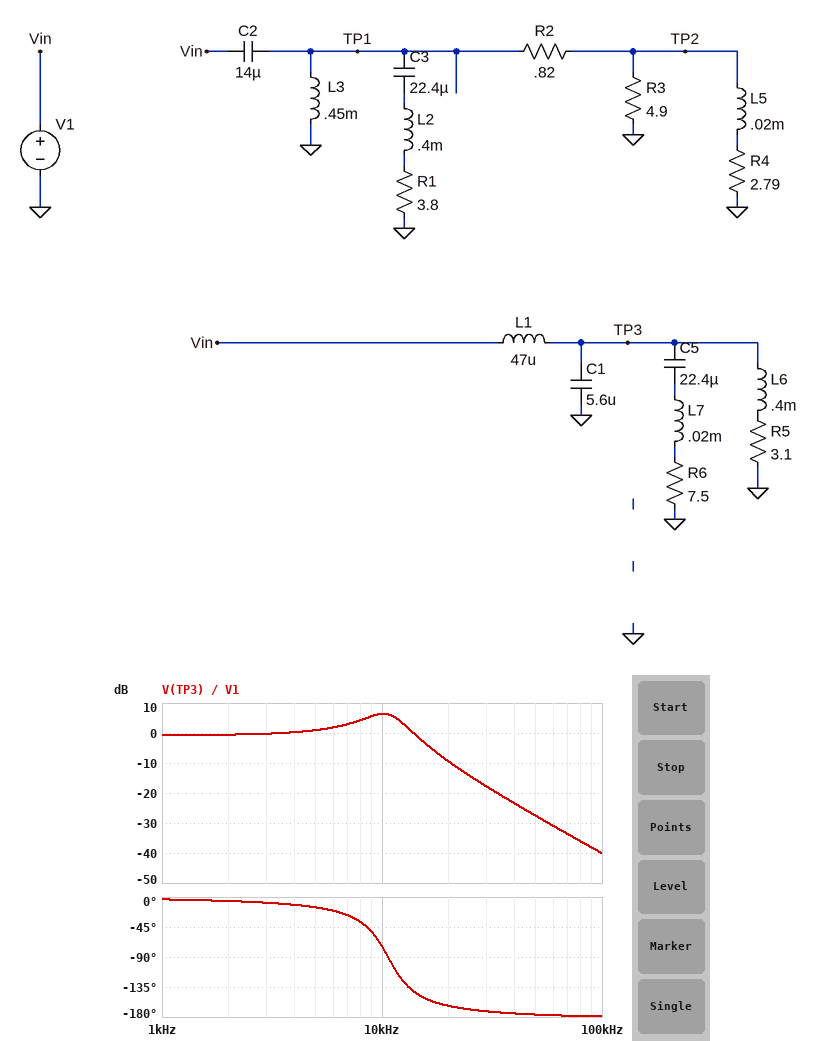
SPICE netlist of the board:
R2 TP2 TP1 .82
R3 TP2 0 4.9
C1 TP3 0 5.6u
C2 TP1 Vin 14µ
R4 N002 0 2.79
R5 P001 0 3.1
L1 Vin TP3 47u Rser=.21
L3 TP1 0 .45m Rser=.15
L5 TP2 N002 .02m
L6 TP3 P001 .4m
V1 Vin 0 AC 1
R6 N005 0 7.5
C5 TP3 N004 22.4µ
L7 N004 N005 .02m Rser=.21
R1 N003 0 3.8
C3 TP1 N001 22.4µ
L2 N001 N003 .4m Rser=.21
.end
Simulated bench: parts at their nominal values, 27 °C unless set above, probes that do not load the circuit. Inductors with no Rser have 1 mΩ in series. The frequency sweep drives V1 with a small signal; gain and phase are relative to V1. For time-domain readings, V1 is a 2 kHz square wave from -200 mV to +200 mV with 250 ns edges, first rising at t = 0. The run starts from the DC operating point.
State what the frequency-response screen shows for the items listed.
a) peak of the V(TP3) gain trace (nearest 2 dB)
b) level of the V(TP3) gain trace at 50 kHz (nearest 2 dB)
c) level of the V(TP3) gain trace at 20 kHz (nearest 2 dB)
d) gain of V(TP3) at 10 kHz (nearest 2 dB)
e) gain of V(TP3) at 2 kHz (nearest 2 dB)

6 dB
-28 dB
-10 dB
6 dB
0 dB
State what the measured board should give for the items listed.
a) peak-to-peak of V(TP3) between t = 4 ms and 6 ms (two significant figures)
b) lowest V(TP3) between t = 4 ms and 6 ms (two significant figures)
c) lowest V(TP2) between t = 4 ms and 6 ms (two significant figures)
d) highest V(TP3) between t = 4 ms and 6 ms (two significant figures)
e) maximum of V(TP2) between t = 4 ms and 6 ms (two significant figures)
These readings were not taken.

720 mV
-360 mV
-340 mV
360 mV
340 mV
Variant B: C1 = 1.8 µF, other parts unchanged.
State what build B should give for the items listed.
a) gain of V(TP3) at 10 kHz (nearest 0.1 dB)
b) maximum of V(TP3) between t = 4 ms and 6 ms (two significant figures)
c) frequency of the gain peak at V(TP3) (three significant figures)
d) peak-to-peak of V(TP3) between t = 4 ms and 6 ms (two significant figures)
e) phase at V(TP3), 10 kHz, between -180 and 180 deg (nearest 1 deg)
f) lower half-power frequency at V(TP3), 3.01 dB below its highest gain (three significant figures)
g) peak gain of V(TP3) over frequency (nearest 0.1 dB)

0.6 dB
290 mV
18.0 kHz
580 mV
-26 deg
6.71 kHz
2.8 dB
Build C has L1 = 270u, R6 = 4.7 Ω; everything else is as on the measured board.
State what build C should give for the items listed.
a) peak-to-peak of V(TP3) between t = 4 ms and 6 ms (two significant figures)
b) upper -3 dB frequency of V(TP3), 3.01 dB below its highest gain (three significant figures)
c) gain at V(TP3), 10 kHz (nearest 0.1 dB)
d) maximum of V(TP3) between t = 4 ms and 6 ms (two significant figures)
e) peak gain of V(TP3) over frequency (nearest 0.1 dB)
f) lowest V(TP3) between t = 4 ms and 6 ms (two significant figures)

350 mV
3.83 kHz
-14.4 dB
170 mV
-0.6 dB
-170 mV
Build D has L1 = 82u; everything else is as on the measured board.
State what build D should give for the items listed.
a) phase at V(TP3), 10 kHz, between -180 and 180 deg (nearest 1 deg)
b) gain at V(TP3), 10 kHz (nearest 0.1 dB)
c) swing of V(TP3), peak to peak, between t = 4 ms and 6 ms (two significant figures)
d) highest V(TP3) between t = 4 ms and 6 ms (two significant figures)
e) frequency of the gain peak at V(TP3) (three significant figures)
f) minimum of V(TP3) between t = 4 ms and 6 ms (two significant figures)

-125 deg
0.7 dB
610 mV
300 mV
7.69 kHz
-300 mV
